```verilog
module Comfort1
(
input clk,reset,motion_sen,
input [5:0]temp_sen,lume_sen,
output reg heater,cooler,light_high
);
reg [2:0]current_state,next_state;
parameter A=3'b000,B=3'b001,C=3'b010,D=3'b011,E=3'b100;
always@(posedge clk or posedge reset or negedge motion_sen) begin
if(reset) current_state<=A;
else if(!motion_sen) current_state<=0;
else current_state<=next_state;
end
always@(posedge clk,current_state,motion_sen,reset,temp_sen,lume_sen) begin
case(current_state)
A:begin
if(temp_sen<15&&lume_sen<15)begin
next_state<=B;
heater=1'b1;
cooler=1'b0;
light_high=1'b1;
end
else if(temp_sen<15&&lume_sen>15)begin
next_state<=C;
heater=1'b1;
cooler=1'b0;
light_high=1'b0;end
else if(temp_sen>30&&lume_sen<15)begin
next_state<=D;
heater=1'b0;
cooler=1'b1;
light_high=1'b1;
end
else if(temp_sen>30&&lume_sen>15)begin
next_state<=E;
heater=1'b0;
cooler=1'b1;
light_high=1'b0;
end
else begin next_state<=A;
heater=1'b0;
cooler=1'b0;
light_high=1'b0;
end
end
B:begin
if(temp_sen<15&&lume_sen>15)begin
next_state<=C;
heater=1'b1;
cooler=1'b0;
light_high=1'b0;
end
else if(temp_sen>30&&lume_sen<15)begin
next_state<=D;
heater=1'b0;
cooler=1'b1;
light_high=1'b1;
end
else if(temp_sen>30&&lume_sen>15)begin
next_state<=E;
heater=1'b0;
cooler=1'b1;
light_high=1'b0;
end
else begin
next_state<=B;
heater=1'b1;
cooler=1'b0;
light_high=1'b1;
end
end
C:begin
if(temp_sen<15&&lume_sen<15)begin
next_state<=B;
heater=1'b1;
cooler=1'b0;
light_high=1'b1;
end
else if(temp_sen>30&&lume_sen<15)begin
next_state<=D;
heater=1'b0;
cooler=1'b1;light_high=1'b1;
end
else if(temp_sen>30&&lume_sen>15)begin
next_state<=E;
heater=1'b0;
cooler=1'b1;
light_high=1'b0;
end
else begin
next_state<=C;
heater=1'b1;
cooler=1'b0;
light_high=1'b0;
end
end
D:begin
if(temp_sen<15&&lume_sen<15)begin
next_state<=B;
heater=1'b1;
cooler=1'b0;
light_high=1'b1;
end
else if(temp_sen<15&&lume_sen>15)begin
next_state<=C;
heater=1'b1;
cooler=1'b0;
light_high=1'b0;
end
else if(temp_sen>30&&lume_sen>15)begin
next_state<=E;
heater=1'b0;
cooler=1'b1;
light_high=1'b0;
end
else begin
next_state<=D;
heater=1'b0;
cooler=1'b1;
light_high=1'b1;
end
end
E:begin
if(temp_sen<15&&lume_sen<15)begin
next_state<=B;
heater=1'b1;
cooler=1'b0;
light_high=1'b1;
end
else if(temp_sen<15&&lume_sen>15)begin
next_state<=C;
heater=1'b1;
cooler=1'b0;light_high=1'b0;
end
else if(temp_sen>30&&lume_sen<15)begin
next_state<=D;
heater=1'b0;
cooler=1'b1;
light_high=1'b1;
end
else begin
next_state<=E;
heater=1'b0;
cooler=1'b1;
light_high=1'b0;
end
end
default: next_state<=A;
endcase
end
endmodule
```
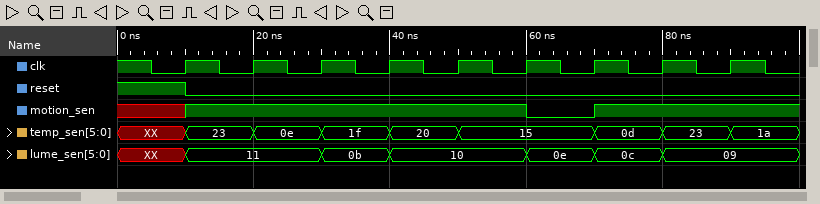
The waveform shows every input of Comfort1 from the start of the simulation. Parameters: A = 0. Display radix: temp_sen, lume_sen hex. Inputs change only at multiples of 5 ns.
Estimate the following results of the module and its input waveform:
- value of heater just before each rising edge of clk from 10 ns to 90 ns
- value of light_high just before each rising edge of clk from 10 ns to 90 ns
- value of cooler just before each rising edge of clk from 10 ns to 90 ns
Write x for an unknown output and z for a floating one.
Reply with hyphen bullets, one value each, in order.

- 0 0 1 0 0 0 0 1 0
- 0 0 0 1 0 0 0 1 1
- 0 1 0 1 1 1 0 0 1
